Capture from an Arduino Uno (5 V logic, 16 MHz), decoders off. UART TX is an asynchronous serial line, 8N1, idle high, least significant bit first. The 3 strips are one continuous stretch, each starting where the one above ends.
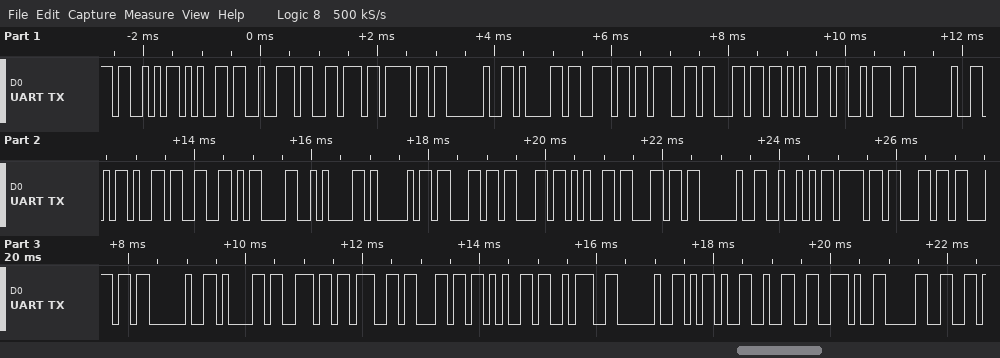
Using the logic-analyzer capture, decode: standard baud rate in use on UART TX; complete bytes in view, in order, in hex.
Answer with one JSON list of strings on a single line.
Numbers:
["9600 baud", "53 65 72 76 6F 20 61 6E 67 6C 65 3A 20 2D 33 0D 0A 41 63 63 65 6C 20 52 6F 6C 6C 20 61 6E 67 6C 65 3A 20 2D 32 2E 30"]
